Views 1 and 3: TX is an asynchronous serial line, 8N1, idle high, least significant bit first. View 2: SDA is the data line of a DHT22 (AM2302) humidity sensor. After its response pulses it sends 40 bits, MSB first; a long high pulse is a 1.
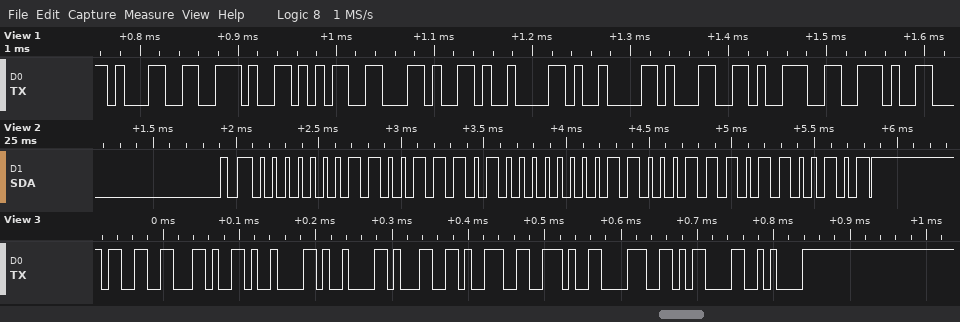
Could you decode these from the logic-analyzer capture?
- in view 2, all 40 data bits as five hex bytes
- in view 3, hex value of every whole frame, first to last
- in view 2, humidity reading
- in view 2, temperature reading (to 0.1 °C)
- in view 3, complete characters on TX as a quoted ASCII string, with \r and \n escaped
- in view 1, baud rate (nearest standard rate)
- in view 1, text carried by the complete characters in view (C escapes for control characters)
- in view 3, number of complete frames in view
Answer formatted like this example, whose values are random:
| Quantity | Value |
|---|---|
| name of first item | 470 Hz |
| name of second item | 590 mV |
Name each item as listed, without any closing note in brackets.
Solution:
| Quantity | Value |
|---|---|
| in view 2, all 40 data bits as five hex bytes | 01 9D 00 C7 65 |
| in view 3, hex value of every whole frame, first to last | 33 2C 09 09 31 39 2E 38 0D 0A |
| in view 2, humidity reading | 41.3 % |
| in view 2, temperature reading | 19.9 °C |
| in view 3, complete characters on TX as a quoted ASCII string, with \r and \n escaped | "3,\t\t19.8\r\n" |
| in view 1, baud rate | 115200 baud |
| in view 1, text carried by the complete characters in view | "1.5,\t\t19." |
| in view 3, number of complete frames in view | 10 |
